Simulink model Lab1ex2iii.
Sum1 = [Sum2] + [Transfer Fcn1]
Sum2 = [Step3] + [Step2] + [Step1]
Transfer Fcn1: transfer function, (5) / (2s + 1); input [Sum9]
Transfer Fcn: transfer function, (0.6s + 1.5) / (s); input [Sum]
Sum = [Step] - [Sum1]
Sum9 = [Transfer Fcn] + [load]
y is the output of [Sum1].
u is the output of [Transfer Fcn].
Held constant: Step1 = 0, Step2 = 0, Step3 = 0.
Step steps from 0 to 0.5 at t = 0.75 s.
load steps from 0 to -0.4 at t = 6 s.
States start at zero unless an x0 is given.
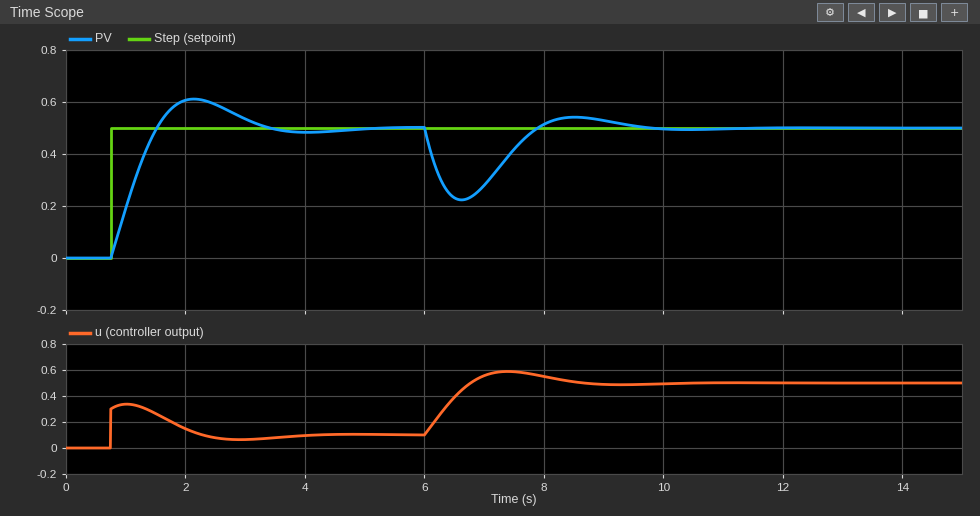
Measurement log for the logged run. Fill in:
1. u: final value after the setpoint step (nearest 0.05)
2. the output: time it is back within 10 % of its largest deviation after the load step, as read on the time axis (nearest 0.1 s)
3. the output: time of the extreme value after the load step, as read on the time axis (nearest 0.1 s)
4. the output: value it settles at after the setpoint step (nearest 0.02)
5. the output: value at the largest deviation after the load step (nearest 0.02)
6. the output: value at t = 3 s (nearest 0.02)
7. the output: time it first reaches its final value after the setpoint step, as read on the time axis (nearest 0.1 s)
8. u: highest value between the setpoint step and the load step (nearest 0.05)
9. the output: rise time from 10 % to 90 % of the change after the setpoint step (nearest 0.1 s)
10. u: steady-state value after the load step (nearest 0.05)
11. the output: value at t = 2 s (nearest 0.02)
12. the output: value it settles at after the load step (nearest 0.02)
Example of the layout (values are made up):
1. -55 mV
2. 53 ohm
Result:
1. 0.10
2. 9.0 s
3. 6.6 s
4. 0.50
5. 0.22
6. 0.54
7. 1.5 s
8. 0.35
9. 0.6 s
10. 0.50
11. 0.60
12. 0.50
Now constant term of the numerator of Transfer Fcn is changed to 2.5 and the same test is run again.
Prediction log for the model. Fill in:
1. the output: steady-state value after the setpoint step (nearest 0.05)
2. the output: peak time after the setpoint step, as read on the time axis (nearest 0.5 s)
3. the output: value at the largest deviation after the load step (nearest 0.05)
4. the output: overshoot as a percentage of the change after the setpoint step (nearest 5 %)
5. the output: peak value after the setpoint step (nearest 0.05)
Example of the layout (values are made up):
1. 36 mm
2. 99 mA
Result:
1. 0.50
2. 2.0 s
3. 0.25
4. 30 %
5. 0.65
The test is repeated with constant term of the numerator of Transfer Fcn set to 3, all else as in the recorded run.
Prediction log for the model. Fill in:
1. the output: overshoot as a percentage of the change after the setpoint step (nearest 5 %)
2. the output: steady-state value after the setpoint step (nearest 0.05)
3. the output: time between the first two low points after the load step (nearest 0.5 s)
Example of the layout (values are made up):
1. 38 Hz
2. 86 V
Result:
1. 35 %
2. 0.50
3. 2.5 s
